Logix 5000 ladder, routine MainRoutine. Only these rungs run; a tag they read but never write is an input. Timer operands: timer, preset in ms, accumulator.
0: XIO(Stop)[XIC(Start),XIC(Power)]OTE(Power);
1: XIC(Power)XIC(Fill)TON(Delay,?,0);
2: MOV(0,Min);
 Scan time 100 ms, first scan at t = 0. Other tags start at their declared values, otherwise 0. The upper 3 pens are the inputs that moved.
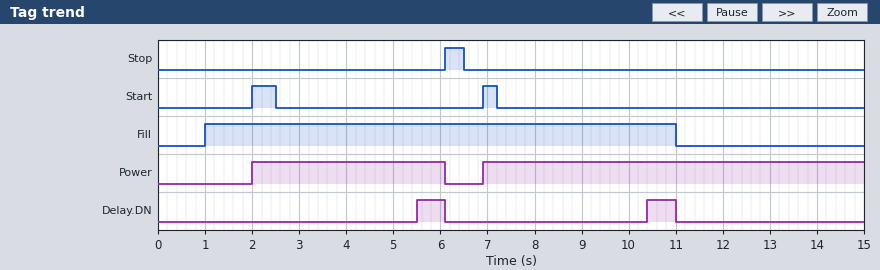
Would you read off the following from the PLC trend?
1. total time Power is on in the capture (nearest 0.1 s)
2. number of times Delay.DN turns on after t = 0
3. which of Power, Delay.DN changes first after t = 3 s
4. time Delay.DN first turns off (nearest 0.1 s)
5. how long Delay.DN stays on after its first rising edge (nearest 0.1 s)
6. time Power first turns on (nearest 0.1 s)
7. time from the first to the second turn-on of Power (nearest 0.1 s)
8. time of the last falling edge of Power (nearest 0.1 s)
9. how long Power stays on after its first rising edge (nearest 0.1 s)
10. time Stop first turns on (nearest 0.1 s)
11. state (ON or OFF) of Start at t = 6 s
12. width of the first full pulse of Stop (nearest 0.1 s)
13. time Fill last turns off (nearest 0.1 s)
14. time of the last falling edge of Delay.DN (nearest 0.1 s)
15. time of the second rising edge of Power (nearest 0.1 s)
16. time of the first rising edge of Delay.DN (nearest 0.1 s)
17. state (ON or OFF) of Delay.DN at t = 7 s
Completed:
12.2 s
2
Delay.DN
6.1 s
0.6 s
2.0 s
4.9 s
6.1 s
4.1 s
6.1 s
OFF
0.4 s
11.0 s
11.0 s
6.9 s
5.5 s
OFF
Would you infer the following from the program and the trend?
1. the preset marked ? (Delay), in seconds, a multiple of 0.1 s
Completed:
3.5 s
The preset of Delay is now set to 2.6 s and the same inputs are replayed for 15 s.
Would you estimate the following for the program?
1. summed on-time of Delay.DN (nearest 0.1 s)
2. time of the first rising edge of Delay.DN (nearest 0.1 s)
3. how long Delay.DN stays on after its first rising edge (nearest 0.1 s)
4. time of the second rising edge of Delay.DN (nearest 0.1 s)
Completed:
3.0 s
4.6 s
1.5 s
9.5 s
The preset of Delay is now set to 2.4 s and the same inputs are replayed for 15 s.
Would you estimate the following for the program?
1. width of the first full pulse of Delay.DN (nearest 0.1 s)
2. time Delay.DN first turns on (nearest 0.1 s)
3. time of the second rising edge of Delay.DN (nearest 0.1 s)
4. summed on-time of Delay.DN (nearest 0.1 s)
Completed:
1.7 s
4.4 s
9.3 s
3.4 s
